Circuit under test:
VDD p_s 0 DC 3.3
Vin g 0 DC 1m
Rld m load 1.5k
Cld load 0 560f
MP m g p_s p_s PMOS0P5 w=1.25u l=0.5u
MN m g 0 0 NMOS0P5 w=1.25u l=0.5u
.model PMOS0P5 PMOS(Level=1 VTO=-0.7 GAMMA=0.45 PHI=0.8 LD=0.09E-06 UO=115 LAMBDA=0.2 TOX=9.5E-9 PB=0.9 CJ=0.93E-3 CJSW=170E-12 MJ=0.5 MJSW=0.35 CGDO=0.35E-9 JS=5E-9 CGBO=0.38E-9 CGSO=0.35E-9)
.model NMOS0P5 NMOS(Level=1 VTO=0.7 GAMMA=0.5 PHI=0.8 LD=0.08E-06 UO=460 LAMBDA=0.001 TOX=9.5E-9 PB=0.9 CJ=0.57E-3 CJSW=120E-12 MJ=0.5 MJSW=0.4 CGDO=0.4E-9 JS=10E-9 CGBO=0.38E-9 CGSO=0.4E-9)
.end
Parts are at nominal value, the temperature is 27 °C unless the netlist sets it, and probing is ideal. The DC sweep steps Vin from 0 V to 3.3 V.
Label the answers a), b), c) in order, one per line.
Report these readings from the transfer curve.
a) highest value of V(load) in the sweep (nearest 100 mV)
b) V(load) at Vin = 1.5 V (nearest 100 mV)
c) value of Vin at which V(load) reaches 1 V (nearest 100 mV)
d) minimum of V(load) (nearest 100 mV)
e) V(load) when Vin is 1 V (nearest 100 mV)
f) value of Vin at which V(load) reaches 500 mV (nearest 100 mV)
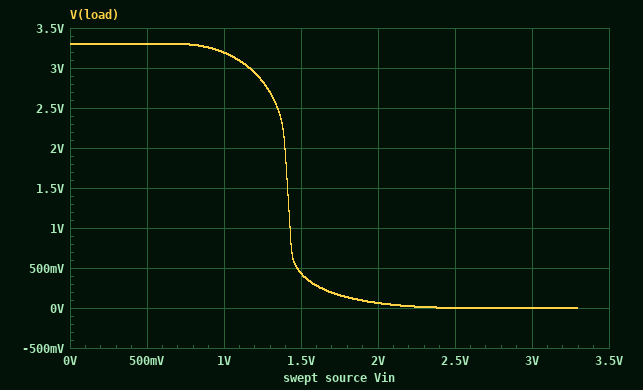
a) 3.3 V
b) 400 mV
c) 1.4 V
d) 0 V
e) 3.2 V
f) 1.5 V
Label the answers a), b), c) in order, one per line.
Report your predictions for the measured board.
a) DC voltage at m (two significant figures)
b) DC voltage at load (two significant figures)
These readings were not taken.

a) 3.3 V
b) 3.3 V
